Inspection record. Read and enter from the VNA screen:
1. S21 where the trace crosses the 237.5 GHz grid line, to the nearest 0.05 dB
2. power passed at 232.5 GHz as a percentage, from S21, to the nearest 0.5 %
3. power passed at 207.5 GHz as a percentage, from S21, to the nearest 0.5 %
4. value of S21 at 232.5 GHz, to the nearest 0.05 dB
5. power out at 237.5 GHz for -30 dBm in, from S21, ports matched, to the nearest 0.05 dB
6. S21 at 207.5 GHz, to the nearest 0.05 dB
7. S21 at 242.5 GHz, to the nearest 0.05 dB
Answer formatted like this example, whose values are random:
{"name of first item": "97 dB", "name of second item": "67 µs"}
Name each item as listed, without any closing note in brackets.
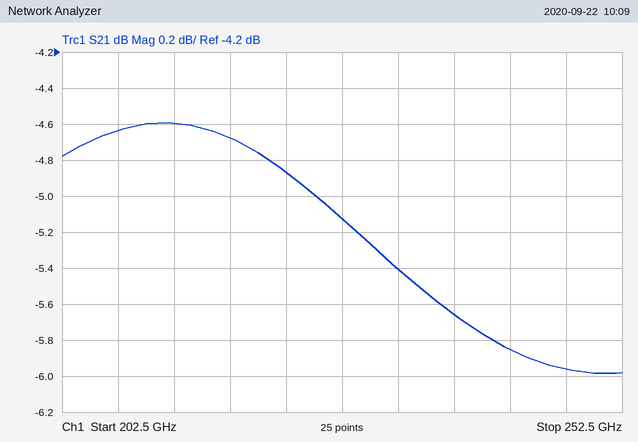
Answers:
{"S21 where the trace crosses the 237.5 GHz grid line, to the nearest 0.05 dB": "-5.65 dB", "power passed at 232.5 GHz as a percentage, from S21, to the nearest 0.5 %": "29.0 %", "power passed at 207.5 GHz as a percentage, from S21, to the nearest 0.5 %": "34.5 %", "value of S21 at 232.5 GHz, to the nearest 0.05 dB": "-5.40 dB", "power out at 237.5 GHz for -30 dBm in, from S21, ports matched, to the nearest 0.05 dB": "-35.65 dBm", "S21 at 207.5 GHz, to the nearest 0.05 dB": "-4.65 dB", "S21 at 242.5 GHz, to the nearest 0.05 dB": "-5.85 dB"}
